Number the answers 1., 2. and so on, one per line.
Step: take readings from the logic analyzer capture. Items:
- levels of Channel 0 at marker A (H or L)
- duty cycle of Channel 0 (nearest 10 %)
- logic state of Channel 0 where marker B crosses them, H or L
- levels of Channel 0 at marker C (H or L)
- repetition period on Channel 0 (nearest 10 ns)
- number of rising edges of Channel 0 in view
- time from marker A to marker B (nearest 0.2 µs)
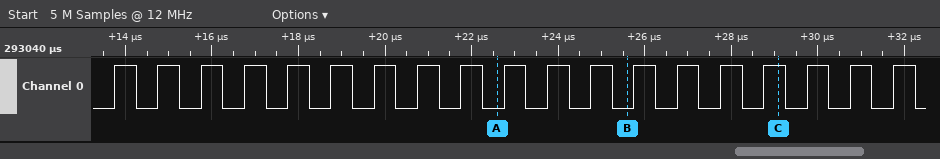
1. Channel 0=L
2. 50 %
3. Channel 0=L
4. Channel 0=H
5. 1000 ns
6. 19
7. 3 µs
